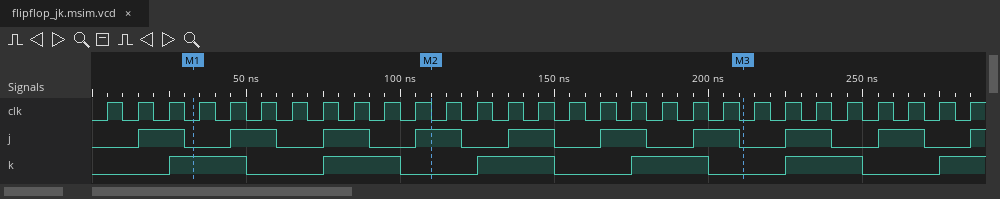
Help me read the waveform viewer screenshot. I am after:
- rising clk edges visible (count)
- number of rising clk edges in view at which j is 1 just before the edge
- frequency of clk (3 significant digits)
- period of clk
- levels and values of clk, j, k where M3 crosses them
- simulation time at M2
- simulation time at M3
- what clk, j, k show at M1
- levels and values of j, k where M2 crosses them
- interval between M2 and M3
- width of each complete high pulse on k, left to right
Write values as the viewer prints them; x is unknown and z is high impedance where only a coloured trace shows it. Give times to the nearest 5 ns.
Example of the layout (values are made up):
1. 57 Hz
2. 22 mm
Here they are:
1. 29
2. 9
3. 100 MHz
4. 10 ns
5. clk=0, j=0, k=0
6. 110 ns
7. 210 ns
8. clk=0, j=0, k=1
9. j=1, k=0
10. 100 ns
11. 25 ns, 25 ns, 25 ns, 25 ns, 25 ns
